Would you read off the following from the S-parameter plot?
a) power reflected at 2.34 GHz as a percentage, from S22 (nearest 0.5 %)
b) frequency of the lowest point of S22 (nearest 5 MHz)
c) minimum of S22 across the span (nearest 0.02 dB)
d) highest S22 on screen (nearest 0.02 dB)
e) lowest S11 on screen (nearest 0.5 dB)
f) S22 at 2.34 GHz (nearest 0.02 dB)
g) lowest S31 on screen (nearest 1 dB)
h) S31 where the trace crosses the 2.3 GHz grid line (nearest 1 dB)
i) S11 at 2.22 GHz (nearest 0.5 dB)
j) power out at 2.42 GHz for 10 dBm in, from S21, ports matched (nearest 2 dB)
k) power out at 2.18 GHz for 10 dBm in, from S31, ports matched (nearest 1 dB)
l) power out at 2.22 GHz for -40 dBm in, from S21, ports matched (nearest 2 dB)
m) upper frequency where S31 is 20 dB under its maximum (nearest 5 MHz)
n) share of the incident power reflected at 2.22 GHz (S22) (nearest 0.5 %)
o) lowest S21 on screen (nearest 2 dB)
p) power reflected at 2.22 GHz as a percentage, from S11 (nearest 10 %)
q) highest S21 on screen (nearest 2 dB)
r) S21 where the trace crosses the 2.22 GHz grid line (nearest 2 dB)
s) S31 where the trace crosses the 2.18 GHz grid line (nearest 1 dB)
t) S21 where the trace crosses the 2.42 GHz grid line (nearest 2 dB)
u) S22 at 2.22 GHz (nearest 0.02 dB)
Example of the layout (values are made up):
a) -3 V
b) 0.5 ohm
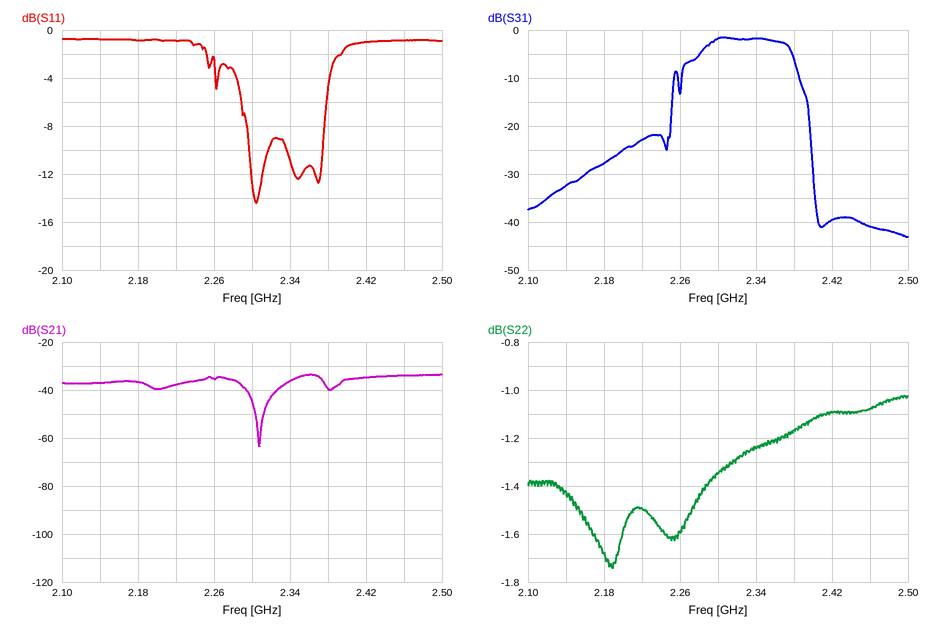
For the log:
a) 75.0 %
b) 2.190 GHz
c) -1.74 dB
d) -1.02 dB
e) -14.5 dB
f) -1.24 dB
g) -43 dB
h) -2 dB
i) -1.0 dB
j) -24 dBm
k) -18 dBm
l) -78 dBm
m) 2.395 GHz
n) 71.0 %
o) -64 dB
p) 80 %
q) -34 dB
r) -38 dB
s) -28 dB
t) -34 dB
u) -1.50 dB
